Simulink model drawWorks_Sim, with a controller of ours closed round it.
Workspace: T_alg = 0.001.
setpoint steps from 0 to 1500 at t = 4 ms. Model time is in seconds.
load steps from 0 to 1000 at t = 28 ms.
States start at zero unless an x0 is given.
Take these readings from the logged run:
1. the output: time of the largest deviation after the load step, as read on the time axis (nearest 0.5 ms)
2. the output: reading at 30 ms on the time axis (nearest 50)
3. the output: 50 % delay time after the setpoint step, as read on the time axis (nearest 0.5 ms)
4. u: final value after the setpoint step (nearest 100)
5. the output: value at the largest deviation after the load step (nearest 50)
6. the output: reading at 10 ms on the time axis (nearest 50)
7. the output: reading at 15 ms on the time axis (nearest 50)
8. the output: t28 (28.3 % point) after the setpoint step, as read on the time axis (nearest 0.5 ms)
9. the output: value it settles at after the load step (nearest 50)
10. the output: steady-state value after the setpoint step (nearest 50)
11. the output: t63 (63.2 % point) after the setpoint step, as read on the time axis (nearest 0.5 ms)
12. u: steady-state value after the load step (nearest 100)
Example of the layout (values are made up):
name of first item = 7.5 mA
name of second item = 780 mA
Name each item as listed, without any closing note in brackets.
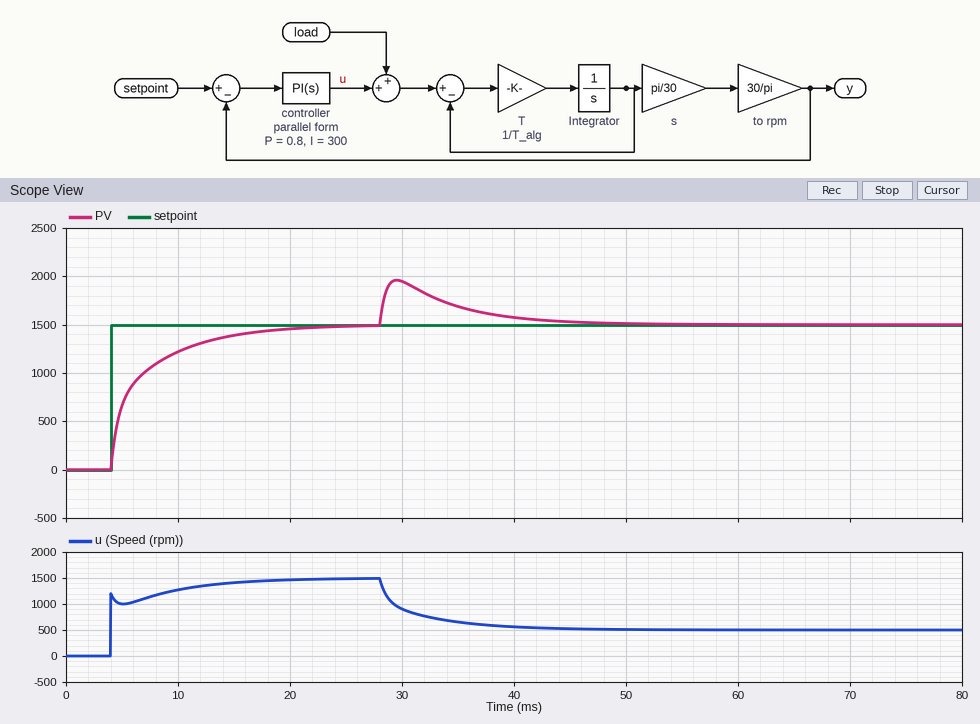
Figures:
the output: time of the largest deviation after the load step, as read on the time axis = 29.5 ms
the output: reading at 30 ms on the time axis = 1950
the output: 50 % delay time after the setpoint step, as read on the time axis = 5.5 ms
u: final value after the setpoint step = 1500
the output: value at the largest deviation after the load step = 1950
the output: reading at 10 ms on the time axis = 1200
the output: reading at 15 ms on the time axis = 1400
the output: t28 (28.3 % point) after the setpoint step, as read on the time axis = 4.5 ms
the output: value it settles at after the load step = 1500
the output: steady-state value after the setpoint step = 1500
the output: t63 (63.2 % point) after the setpoint step, as read on the time axis = 6.5 ms
u: steady-state value after the load step = 500
